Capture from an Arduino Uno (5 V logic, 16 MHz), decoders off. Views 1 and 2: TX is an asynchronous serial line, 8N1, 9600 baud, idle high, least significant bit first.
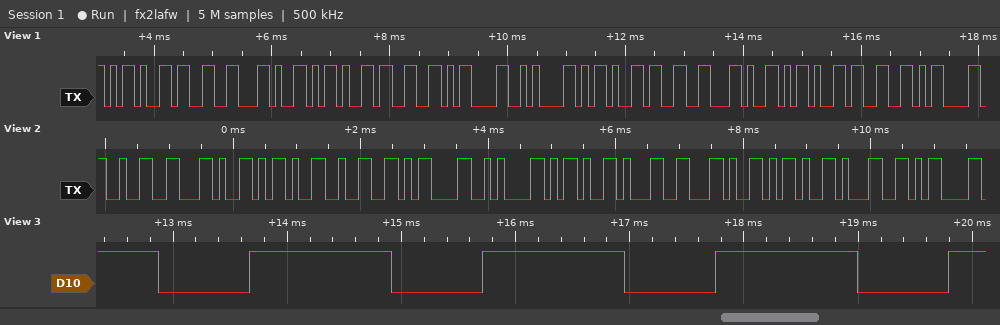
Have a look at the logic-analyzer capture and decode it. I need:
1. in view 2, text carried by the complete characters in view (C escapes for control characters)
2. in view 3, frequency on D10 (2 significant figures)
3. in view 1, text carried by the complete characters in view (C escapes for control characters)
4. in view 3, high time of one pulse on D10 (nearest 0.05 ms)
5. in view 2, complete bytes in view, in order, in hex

"2,-2\r\n-1,-1\r"
490 Hz
"-3,-3\r\n-3,-3\r"
1.25 ms
32 2C 2D 32 0D 0A 2D 31 2C 2D 31 0D
